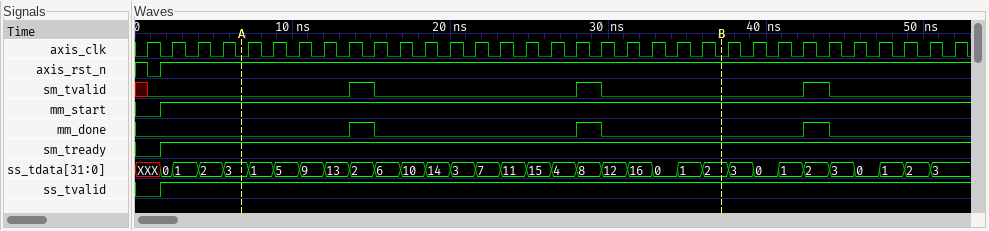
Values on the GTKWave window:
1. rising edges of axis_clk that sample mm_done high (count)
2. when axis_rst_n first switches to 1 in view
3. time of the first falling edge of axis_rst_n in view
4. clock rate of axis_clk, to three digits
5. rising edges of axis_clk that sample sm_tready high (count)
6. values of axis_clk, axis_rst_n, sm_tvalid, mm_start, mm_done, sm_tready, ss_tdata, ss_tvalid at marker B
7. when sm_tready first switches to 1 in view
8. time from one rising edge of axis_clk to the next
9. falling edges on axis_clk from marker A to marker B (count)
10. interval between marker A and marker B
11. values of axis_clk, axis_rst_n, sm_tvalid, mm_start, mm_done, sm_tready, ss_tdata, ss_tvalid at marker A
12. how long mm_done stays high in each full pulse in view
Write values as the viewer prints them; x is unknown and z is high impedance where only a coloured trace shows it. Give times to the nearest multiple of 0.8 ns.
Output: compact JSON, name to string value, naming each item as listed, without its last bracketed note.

{"rising edges of axis_clk that sample mm_done high": "3", "when axis_rst_n first switches to 1 in view": "1.6 ns", "time of the first falling edge of axis_rst_n in view": "0.8 ns", "clock rate of axis_clk, to three digits": "625 MHz", "rising edges of axis_clk that sample sm_tready high": "32", "values of axis_clk, axis_rst_n, sm_tvalid, mm_start, mm_done, sm_tready, ss_tdata, ss_tvalid at marker B": "axis_clk=0, axis_rst_n=1, sm_tvalid=0, mm_start=1, mm_done=0, sm_tready=1, ss_tdata=2, ss_tvalid=1", "when sm_tready first switches to 1 in view": "1.6 ns", "time from one rising edge of axis_clk to the next": "1.6 ns", "falling edges on axis_clk from marker A to marker B": "19", "interval between marker A and marker B": "30.4 ns", "values of axis_clk, axis_rst_n, sm_tvalid, mm_start, mm_done, sm_tready, ss_tdata, ss_tvalid at marker A": "axis_clk=0, axis_rst_n=1, sm_tvalid=0, mm_start=1, mm_done=0, sm_tready=1, ss_tdata=3, ss_tvalid=1", "how long mm_done stays high in each full pulse in view": "1.6 ns, 1.6 ns, 1.6 ns"}
